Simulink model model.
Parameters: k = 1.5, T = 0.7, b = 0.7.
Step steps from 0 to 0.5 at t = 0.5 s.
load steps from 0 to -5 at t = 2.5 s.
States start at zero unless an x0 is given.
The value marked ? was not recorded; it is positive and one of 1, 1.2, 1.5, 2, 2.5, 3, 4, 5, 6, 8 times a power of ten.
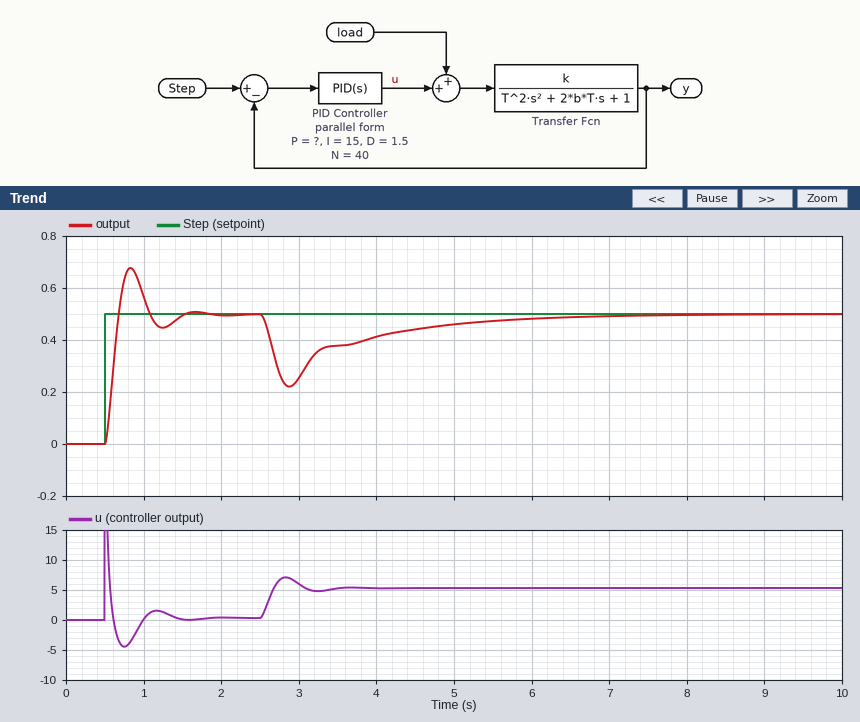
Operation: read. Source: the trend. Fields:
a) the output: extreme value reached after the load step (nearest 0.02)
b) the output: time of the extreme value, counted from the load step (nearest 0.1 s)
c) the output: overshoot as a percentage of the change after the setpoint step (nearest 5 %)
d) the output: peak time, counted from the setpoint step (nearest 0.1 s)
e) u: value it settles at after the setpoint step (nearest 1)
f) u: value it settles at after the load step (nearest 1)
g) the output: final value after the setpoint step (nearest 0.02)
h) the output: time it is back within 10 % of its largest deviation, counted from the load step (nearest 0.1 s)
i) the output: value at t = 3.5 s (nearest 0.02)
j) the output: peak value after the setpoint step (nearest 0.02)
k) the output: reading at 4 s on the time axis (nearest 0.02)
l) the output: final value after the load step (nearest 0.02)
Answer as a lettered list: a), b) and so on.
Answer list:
a) 0.22
b) 0.4 s
c) 35 %
d) 0.3 s
e) 0
f) 5
g) 0.50
h) 3.0 s
i) 0.38
j) 0.68
k) 0.42
l) 0.50
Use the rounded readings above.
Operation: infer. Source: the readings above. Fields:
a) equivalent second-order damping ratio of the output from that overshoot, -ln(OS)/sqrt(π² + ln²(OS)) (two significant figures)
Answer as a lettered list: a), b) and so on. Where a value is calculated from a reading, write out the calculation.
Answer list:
a) ln(0.35) = -1.050; 1.050 / sqrt(9.870 + 1.102) = 0.32
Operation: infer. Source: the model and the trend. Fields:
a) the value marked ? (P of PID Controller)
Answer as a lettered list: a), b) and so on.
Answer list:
a) 20
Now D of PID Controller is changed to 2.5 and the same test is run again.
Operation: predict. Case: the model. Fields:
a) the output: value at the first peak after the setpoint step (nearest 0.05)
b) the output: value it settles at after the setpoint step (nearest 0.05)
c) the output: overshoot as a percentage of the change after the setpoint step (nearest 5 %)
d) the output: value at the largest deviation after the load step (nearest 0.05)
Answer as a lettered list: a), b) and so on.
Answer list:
a) 0.60
b) 0.50
c) 25 %
d) 0.25
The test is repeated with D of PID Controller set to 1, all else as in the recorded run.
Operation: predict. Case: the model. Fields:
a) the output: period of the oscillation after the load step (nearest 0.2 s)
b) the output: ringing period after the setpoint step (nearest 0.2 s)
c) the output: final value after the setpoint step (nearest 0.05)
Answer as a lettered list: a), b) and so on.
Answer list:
a) 0.8 s
b) 0.8 s
c) 0.50
